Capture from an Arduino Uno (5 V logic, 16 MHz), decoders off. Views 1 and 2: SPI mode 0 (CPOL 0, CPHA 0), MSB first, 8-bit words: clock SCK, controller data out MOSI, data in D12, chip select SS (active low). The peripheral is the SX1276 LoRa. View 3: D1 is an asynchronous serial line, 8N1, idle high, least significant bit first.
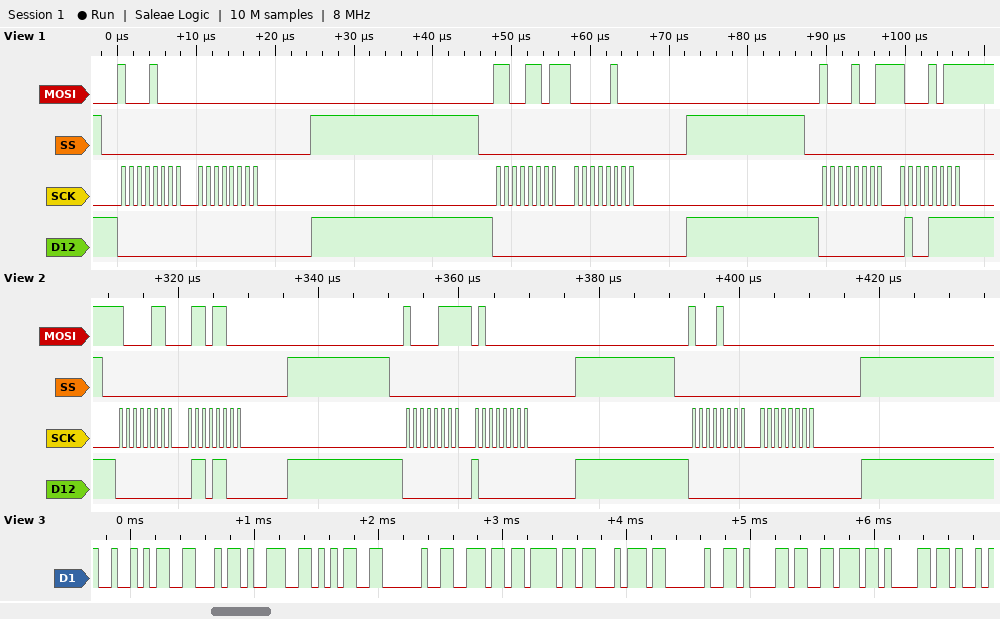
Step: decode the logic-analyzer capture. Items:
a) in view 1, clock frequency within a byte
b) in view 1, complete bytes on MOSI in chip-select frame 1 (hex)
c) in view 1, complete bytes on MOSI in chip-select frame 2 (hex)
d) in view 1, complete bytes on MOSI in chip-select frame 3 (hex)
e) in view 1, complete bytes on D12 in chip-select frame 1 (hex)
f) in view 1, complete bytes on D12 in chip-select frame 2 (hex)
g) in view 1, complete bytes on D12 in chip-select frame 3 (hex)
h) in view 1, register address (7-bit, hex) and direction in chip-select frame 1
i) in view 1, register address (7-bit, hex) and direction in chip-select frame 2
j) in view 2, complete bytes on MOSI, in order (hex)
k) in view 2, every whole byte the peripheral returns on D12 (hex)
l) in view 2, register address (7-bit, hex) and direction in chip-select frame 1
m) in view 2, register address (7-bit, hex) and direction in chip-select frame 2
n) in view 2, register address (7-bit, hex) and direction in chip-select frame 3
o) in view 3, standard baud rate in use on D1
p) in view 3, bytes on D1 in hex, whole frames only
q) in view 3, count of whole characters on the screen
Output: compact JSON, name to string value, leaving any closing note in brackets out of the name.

{"in view 1, clock frequency within a byte": "1 MHz", "in view 1, complete bytes on MOSI in chip-select frame 1": "0x88 0x00", "in view 1, complete bytes on MOSI in chip-select frame 2": "0xCD 0x04", "in view 1, complete bytes on MOSI in chip-select frame 3": "0x89 0x8B", "in view 1, complete bytes on D12 in chip-select frame 1": "0x00 0x00", "in view 1, complete bytes on D12 in chip-select frame 2": "0x00 0x00", "in view 1, complete bytes on D12 in chip-select frame 3": "0x00 0x4F", "in view 1, register address (7-bit, hex) and direction in chip-select frame 1": "0x08 write", "in view 1, register address (7-bit, hex) and direction in chip-select frame 2": "0x4D write", "in view 2, complete bytes on MOSI, in order": "86 6C 87 40 88 00", "in view 2, every whole byte the peripheral returns on D12": "00 6C 00 80 00 00", "in view 2, register address (7-bit, hex) and direction in chip-select frame 1": "0x06 write", "in view 2, register address (7-bit, hex) and direction in chip-select frame 2": "0x07 write", "in view 2, register address (7-bit, hex) and direction in chip-select frame 3": "0x08 write", "in view 3, standard baud rate in use on D1": "19200 baud", "in view 3, bytes on D1 in hex, whole frames only": "52 46 39 35 20 6E 6F 74 20 61 76 61", "in view 3, count of whole characters on the screen": "12"}
